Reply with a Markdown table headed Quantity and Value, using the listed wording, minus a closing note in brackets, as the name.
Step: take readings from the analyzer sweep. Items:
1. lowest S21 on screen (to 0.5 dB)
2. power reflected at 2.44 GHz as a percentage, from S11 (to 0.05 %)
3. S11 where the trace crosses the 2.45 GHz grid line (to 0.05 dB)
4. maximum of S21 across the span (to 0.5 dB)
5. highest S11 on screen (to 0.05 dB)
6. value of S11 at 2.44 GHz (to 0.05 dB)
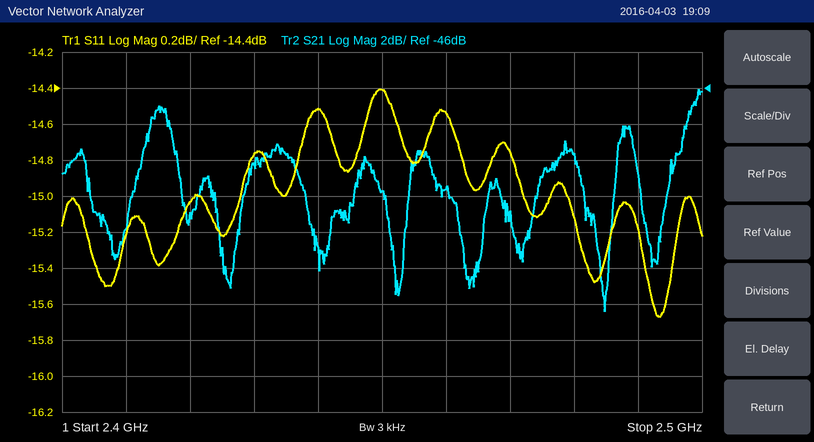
| Quantity | Value |
|---|---|
| lowest S21 on screen | -58.5 dB |
| power reflected at 2.44 GHz as a percentage, from S11 | 3.55 % |
| S11 where the trace crosses the 2.45 GHz grid line | -14.40 dB |
| maximum of S21 across the span | -46.0 dB |
| highest S11 on screen | -14.40 dB |
| value of S11 at 2.44 GHz | -14.50 dB |
